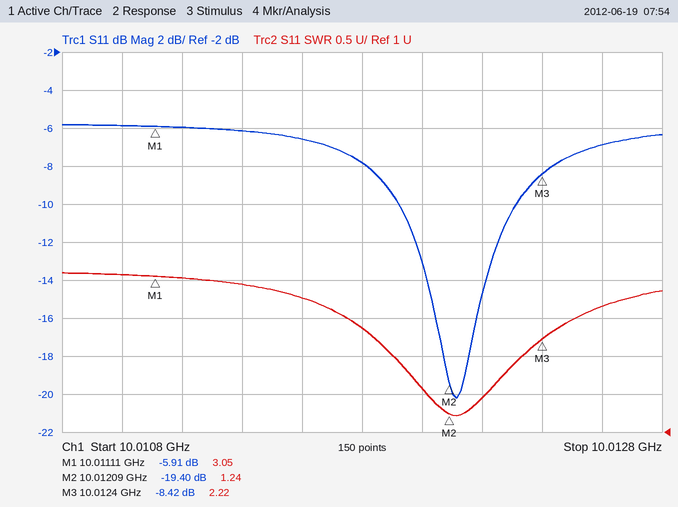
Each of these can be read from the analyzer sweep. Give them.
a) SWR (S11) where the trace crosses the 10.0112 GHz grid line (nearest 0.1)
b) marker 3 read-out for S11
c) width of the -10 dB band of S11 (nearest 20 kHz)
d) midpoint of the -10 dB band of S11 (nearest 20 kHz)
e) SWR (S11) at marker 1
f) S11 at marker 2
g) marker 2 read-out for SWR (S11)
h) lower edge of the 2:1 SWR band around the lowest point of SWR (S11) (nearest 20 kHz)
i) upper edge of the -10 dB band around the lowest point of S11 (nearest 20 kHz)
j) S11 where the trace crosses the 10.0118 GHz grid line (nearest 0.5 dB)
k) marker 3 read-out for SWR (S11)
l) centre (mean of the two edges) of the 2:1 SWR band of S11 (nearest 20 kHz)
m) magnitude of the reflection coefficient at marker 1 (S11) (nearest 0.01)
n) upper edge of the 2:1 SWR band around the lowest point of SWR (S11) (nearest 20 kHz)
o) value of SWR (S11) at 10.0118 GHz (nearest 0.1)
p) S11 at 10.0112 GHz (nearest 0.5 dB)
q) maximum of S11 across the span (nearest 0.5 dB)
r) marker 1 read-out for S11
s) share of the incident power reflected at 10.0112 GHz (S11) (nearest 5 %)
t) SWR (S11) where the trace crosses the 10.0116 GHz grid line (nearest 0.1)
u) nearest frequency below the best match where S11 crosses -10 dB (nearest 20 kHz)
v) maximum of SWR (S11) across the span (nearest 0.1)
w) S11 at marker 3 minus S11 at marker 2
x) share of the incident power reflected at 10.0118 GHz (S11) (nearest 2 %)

3.0
-8.42 dB
400 kHz
10.01212 GHz
3.05
-19.40 dB
1.24
10.01190 GHz
10.01232 GHz
-8.0 dB
2.22
10.01212 GHz
0.51
10.01234 GHz
2.4
-6.0 dB
-6.0 dB
-5.91 dB
25 %
2.8
10.01192 GHz
3.1
10.98 dB
16 %
